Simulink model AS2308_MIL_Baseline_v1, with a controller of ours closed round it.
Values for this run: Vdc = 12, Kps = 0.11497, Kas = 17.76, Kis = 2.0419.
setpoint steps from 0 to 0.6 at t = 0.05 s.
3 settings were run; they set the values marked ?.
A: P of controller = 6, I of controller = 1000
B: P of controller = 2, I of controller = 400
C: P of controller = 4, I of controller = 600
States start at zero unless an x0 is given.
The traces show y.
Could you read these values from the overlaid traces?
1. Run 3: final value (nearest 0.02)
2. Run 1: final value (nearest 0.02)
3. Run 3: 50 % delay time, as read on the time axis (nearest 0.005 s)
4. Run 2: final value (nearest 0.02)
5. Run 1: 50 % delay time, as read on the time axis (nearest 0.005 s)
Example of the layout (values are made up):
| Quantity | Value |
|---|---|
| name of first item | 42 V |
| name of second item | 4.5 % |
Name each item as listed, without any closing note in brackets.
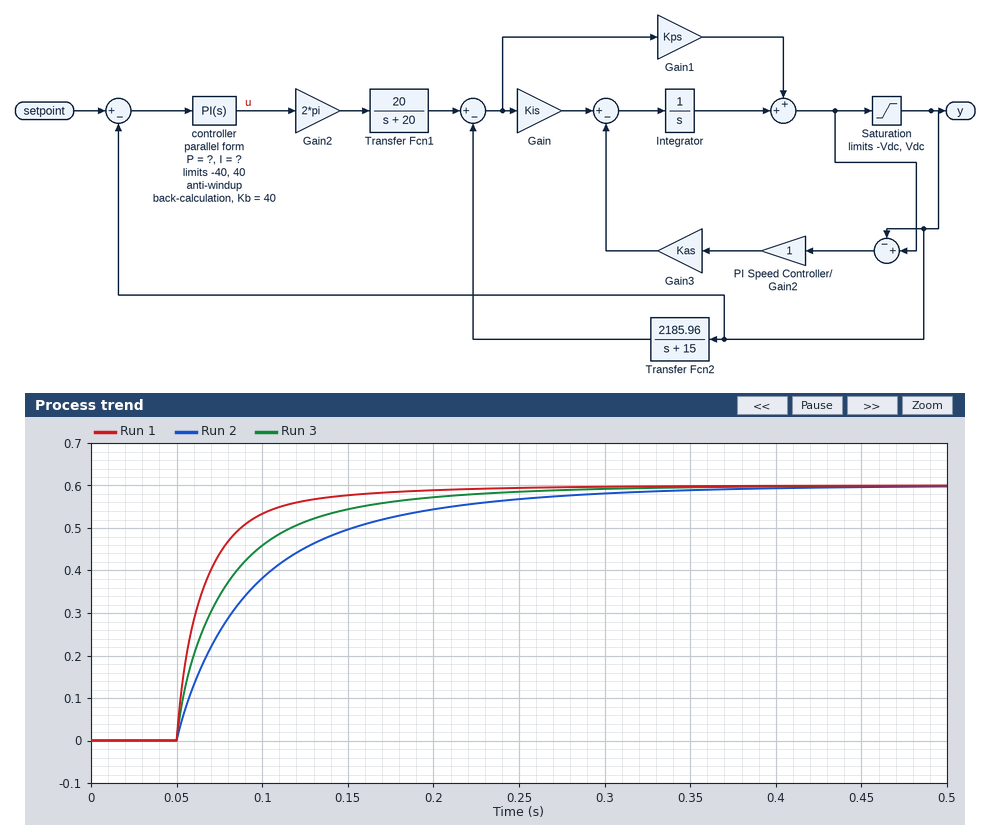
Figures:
| Quantity | Value |
|---|---|
| Run 3: final value | 0.60 |
| Run 1: final value | 0.60 |
| Run 3: 50 % delay time, as read on the time axis | 0.070 s |
| Run 2: final value | 0.60 |
| Run 1: 50 % delay time, as read on the time axis | 0.060 s |
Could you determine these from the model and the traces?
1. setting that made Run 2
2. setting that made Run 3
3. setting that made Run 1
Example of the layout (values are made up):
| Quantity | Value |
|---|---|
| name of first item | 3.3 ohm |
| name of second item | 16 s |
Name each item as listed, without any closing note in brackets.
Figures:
| Quantity | Value |
|---|---|
| setting that made Run 2 | B |
| setting that made Run 3 | C |
| setting that made Run 1 | A |
